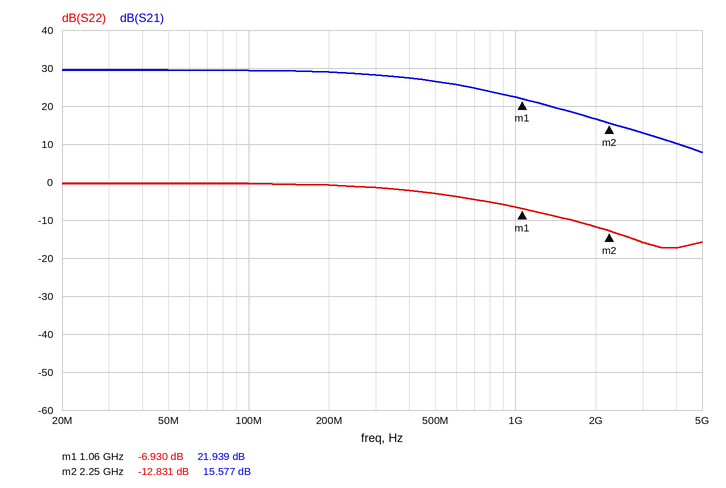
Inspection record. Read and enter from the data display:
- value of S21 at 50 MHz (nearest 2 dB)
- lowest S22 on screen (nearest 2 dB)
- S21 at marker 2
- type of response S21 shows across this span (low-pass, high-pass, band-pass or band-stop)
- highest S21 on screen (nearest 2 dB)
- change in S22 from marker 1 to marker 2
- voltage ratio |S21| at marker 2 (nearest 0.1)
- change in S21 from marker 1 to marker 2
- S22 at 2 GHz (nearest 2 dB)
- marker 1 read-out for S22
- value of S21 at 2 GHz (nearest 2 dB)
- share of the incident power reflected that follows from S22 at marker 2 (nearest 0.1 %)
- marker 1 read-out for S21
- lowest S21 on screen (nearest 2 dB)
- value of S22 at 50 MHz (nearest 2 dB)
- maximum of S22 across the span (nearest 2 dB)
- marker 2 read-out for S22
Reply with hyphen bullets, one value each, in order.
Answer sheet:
- 30 dB
- -18 dB
- 15.577 dB
- low-pass
- 30 dB
- -5.901 dB
- 6.0
- -6.362 dB
- -12 dB
- -6.930 dB
- 16 dB
- 5.2 %
- 21.939 dB
- 8 dB
- 0 dB
- 0 dB
- -12.831 dB
